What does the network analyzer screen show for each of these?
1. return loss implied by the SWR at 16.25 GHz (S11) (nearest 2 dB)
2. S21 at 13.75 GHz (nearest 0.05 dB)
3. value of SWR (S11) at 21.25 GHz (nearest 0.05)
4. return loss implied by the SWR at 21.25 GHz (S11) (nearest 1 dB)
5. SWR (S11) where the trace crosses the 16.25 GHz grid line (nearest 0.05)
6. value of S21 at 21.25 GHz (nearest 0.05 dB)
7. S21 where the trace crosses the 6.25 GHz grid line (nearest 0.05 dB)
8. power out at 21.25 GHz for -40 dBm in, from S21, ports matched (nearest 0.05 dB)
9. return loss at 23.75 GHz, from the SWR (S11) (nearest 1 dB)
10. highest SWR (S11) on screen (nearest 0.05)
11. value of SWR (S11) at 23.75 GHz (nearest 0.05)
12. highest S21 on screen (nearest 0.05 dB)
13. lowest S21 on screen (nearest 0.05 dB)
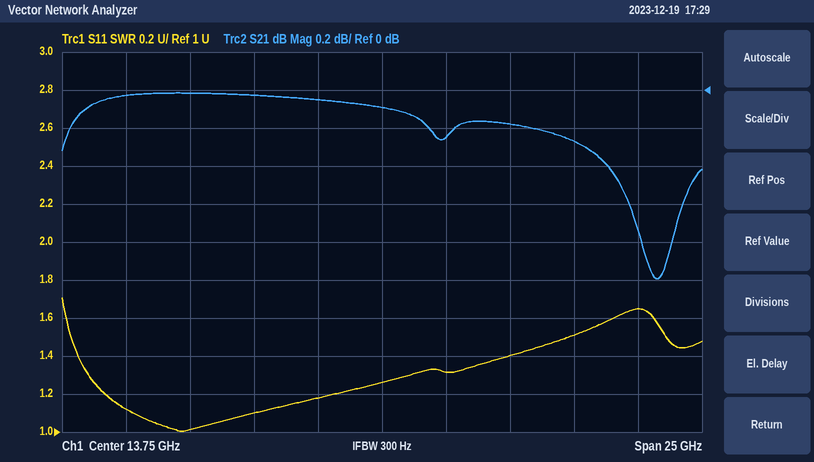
18 dB
-0.10 dB
1.50
14 dB
1.30
-0.25 dB
0.00 dB
-40.25 dBm
12 dB
1.70
1.65
0.00 dB
-1.00 dB
